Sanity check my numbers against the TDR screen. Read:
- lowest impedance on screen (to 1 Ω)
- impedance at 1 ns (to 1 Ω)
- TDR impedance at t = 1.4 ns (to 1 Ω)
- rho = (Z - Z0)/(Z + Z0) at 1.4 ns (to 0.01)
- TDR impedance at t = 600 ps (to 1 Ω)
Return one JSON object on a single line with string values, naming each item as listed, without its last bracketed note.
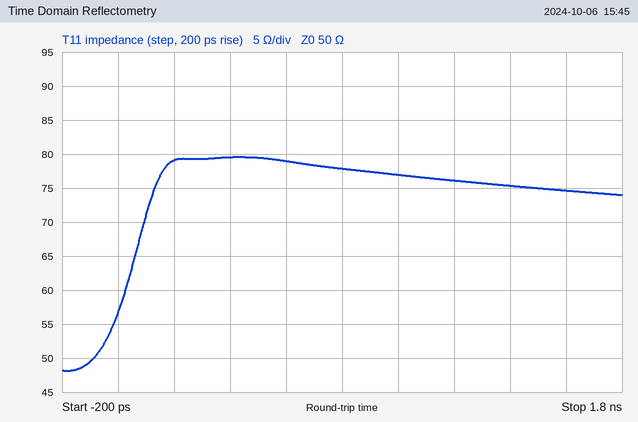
{"lowest impedance on screen": "48 Ω", "impedance at 1 ns": "77 Ω", "TDR impedance at t = 1.4 ns": "75 Ω", "rho = (Z - Z0)/(Z + Z0) at 1.4 ns": "+0.20", "TDR impedance at t = 600 ps": "79 Ω"}
